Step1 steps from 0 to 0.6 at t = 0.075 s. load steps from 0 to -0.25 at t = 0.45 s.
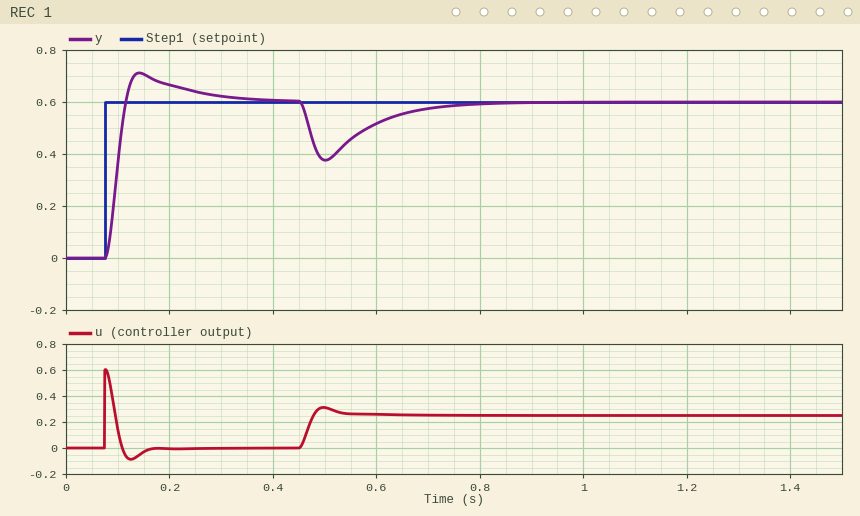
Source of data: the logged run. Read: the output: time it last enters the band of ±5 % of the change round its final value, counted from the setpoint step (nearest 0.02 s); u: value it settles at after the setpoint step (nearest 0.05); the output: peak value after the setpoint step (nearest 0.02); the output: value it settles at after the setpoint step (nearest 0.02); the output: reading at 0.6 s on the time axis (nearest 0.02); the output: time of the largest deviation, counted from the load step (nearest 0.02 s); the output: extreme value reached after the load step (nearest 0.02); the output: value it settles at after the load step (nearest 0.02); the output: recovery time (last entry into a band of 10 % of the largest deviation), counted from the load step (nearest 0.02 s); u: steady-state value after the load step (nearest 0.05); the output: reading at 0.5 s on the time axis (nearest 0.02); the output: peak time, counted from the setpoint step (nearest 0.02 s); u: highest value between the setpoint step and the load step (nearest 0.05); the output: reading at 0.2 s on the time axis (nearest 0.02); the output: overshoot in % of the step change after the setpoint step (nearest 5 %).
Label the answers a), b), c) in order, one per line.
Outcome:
a) 0.20 s
b) 0.00
c) 0.72
d) 0.60
e) 0.52
f) 0.06 s
g) 0.38
h) 0.60
i) 0.26 s
j) 0.25
k) 0.38
l) 0.06 s
m) 0.60
n) 0.66
o) 20 %
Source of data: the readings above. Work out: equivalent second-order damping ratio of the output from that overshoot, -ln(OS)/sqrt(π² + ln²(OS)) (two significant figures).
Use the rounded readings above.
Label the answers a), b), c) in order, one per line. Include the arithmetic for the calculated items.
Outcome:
a) ln(0.2) = -1.609; 1.609 / sqrt(9.870 + 2.590) = 0.46
